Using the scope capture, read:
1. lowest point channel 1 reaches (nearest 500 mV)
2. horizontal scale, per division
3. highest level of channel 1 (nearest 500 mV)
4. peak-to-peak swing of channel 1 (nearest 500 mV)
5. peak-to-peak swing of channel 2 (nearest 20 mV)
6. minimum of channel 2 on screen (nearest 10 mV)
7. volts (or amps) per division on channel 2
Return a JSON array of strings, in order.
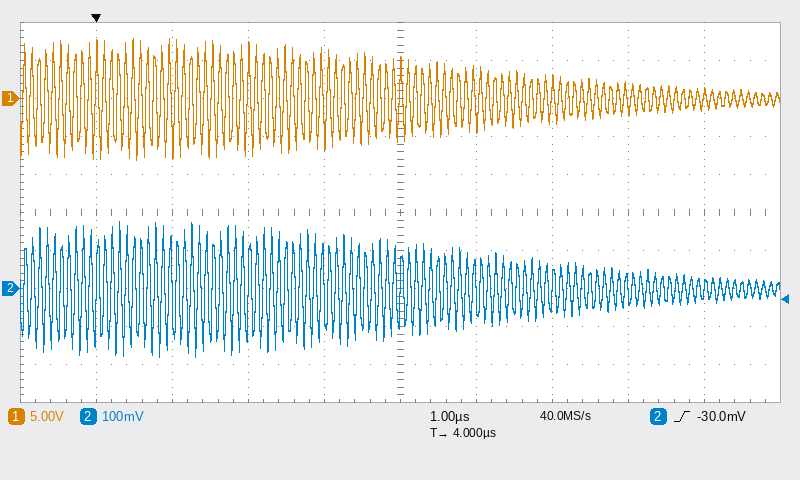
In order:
["-8.0 V", "1 µs", "8.0 V", "16.0 V", "360 mV", "-180 mV", "100 mV"]
